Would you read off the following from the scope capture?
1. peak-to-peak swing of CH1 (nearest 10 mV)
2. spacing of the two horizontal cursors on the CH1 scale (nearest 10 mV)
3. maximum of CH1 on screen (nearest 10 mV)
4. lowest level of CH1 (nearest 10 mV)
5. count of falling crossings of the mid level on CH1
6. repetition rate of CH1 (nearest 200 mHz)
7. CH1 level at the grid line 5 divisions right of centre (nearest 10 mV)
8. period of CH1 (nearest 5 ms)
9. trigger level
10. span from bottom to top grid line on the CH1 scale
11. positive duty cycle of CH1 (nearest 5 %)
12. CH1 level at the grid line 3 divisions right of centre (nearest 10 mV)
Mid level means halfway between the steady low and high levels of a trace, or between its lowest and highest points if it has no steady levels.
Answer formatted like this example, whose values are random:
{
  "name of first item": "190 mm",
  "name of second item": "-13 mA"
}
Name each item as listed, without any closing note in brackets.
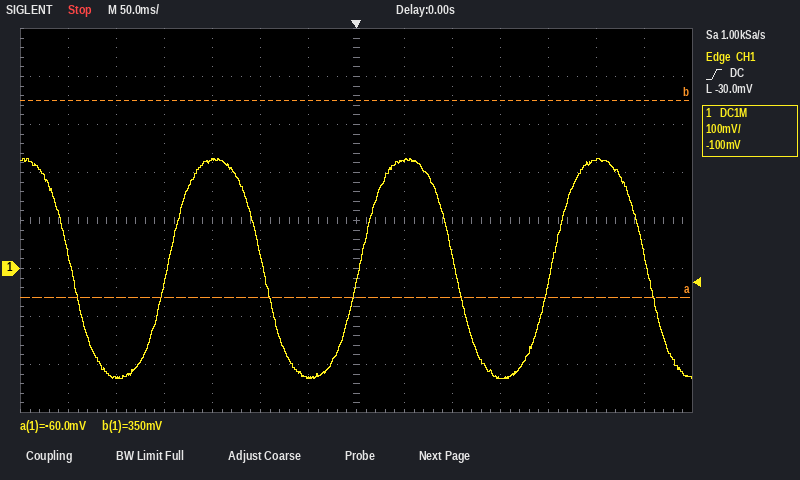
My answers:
{
  "peak-to-peak swing of CH1": "460 mV",
  "spacing of the two horizontal cursors on the CH1 scale": "410 mV",
  "maximum of CH1 on screen": "230 mV",
  "lowest level of CH1": "-230 mV",
  "count of falling crossings of the mid level on CH1": "4",
  "repetition rate of CH1": "5.0 Hz",
  "CH1 level at the grid line 5 divisions right of centre": "230 mV",
  "period of CH1": "200 ms",
  "trigger level": "-30.0 mV",
  "span from bottom to top grid line on the CH1 scale": "800 mV",
  "positive duty cycle of CH1": "50 %",
  "CH1 level at the grid line 3 divisions right of centre": "-230 mV"
}
